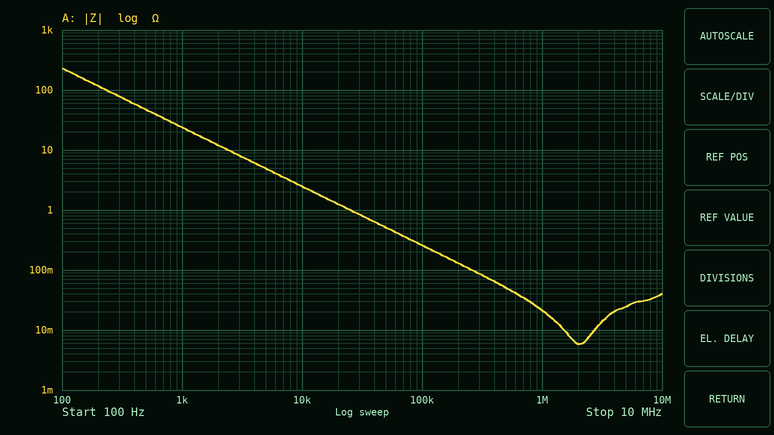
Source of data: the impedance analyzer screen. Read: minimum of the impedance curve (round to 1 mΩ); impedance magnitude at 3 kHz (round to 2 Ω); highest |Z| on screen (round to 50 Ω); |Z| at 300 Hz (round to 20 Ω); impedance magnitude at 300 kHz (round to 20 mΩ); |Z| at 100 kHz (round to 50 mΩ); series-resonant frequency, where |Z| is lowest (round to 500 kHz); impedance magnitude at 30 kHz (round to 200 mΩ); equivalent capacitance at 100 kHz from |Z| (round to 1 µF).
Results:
6 mΩ
8 Ω
250 Ω
80 Ω
80 mΩ
250 mΩ
2.0 MHz
800 mΩ
6 µF
